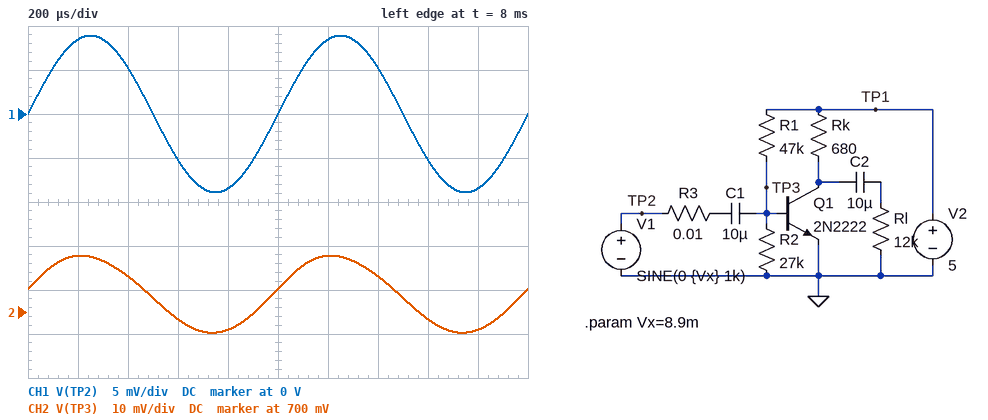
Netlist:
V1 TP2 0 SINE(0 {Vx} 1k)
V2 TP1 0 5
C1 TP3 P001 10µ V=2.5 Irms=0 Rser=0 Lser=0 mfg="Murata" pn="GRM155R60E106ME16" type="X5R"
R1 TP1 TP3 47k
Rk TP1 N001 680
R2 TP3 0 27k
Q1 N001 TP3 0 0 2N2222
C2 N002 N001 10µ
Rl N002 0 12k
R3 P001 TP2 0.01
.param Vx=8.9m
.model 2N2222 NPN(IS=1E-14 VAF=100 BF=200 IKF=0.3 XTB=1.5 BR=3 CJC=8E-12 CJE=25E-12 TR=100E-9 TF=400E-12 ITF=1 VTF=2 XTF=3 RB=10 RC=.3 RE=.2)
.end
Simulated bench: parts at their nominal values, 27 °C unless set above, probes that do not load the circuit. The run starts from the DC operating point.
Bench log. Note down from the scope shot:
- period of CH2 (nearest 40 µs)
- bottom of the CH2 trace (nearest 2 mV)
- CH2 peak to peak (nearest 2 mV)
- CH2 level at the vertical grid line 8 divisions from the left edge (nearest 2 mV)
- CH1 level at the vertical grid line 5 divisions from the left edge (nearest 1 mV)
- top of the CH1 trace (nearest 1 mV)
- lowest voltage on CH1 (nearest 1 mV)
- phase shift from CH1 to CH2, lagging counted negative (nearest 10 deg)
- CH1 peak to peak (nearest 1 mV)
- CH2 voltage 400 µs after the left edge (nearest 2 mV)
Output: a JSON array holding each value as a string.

["1.00 ms", "696 mV", "18 mV", "698 mV", "0 V", "9 mV", "-9 mV", "10 deg", "18 mV", "708 mV"]
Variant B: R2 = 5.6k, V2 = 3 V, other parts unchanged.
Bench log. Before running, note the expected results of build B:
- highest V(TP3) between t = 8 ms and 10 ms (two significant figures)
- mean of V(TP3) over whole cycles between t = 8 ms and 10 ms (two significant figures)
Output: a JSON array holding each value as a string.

["330 mV", "320 mV"]
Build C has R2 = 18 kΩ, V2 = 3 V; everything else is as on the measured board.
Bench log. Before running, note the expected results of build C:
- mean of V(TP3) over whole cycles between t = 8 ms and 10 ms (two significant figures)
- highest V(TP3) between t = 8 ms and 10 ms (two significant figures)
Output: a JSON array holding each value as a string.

["680 mV", "690 mV"]
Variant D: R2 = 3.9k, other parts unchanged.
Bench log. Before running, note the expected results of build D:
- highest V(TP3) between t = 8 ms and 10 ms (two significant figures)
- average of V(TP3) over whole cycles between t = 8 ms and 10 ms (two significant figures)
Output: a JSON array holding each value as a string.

["390 mV", "380 mV"]
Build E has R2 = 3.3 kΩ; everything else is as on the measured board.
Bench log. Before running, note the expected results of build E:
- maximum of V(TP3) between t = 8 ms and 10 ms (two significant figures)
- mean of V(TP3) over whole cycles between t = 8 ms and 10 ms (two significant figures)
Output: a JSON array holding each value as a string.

["340 mV", "330 mV"]
